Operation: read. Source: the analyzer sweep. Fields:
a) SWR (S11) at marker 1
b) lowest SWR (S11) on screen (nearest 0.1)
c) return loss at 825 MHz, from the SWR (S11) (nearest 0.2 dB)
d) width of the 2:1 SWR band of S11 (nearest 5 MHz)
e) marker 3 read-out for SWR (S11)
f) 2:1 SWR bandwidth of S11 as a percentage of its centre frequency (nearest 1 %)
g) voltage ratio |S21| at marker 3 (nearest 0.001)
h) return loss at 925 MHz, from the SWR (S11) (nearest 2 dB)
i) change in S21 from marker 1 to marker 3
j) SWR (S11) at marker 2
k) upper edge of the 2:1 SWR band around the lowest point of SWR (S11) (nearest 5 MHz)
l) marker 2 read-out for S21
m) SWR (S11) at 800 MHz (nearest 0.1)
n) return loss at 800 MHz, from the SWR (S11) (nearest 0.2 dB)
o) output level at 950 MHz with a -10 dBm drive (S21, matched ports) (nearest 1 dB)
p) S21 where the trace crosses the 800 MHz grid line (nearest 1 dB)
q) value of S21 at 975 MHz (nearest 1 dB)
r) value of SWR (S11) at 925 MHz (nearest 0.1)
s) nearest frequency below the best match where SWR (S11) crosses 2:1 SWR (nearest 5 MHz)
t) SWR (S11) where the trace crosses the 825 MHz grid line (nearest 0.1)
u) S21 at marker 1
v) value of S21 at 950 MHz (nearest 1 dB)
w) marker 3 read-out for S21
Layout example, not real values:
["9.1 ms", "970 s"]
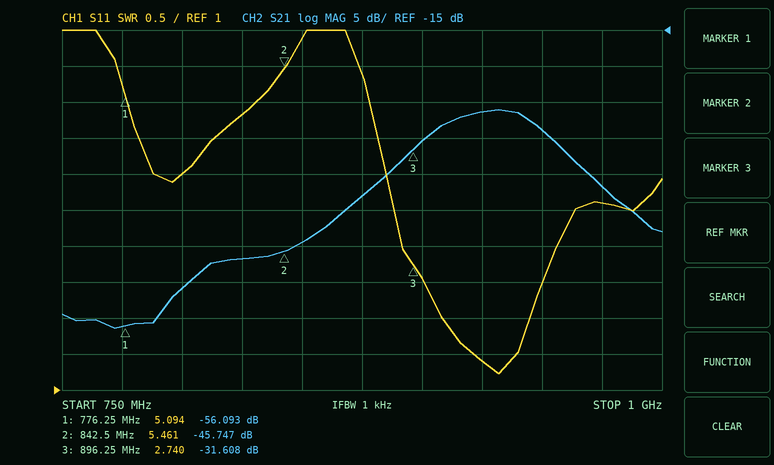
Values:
["5.094", "1.2", "3.6 dB", "35 MHz", "2.740", "4 %", "0.026", "16 dB", "24.485 dB", "5.461", "945 MHz", "-45.747 dB", "4.0", "4.4 dB", "-39 dBm", "-51 dB", "-37 dB", "1.4", "910 MHz", "4.8", "-56.093 dB", "-29 dB", "-31.608 dB"]
